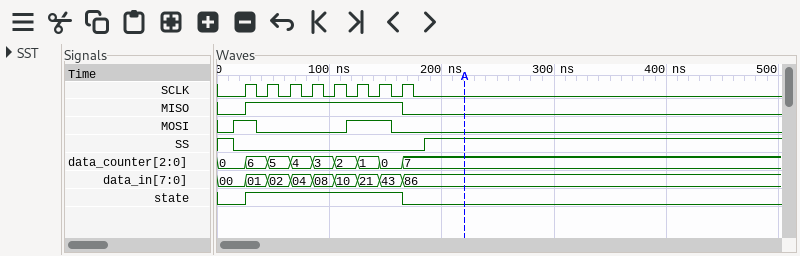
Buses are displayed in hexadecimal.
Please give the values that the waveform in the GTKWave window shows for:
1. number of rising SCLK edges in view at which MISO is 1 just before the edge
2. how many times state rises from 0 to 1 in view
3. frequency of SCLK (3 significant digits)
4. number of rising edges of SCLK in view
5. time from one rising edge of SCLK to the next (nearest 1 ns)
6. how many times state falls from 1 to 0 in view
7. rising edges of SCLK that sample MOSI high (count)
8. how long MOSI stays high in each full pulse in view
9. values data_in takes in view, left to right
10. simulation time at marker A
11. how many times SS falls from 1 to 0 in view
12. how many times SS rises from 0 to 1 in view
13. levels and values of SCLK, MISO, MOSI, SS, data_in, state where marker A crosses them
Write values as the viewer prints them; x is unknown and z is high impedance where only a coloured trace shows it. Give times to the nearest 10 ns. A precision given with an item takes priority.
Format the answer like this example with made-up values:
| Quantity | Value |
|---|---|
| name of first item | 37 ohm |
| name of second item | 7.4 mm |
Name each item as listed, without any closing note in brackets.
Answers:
| Quantity | Value |
|---|---|
| number of rising SCLK edges in view at which MISO is 1 just before the edge | 7 |
| how many times state rises from 0 to 1 in view | 1 |
| frequency of SCLK | 50.0 MHz |
| number of rising edges of SCLK in view | 8 |
| time from one rising edge of SCLK to the next | 20 ns |
| how many times state falls from 1 to 0 in view | 1 |
| rising edges of SCLK that sample MOSI high | 3 |
| how long MOSI stays high in each full pulse in view | 20 ns, 40 ns |
| values data_in takes in view, left to right | 00, 01, 02, 04, 08, 10, 21, 43, 86 |
| simulation time at marker A | 220 ns |
| how many times SS falls from 1 to 0 in view | 1 |
| how many times SS rises from 0 to 1 in view | 1 |
| levels and values of SCLK, MISO, MOSI, SS, data_in, state where marker A crosses them | SCLK=0, MISO=0, MOSI=0, SS=1, data_in=86, state=0 |
